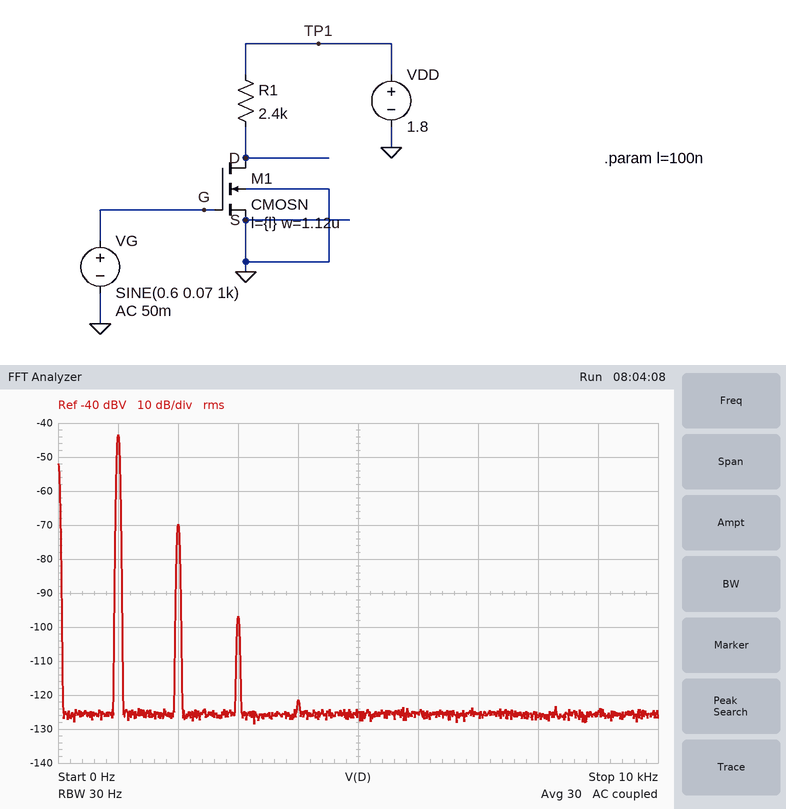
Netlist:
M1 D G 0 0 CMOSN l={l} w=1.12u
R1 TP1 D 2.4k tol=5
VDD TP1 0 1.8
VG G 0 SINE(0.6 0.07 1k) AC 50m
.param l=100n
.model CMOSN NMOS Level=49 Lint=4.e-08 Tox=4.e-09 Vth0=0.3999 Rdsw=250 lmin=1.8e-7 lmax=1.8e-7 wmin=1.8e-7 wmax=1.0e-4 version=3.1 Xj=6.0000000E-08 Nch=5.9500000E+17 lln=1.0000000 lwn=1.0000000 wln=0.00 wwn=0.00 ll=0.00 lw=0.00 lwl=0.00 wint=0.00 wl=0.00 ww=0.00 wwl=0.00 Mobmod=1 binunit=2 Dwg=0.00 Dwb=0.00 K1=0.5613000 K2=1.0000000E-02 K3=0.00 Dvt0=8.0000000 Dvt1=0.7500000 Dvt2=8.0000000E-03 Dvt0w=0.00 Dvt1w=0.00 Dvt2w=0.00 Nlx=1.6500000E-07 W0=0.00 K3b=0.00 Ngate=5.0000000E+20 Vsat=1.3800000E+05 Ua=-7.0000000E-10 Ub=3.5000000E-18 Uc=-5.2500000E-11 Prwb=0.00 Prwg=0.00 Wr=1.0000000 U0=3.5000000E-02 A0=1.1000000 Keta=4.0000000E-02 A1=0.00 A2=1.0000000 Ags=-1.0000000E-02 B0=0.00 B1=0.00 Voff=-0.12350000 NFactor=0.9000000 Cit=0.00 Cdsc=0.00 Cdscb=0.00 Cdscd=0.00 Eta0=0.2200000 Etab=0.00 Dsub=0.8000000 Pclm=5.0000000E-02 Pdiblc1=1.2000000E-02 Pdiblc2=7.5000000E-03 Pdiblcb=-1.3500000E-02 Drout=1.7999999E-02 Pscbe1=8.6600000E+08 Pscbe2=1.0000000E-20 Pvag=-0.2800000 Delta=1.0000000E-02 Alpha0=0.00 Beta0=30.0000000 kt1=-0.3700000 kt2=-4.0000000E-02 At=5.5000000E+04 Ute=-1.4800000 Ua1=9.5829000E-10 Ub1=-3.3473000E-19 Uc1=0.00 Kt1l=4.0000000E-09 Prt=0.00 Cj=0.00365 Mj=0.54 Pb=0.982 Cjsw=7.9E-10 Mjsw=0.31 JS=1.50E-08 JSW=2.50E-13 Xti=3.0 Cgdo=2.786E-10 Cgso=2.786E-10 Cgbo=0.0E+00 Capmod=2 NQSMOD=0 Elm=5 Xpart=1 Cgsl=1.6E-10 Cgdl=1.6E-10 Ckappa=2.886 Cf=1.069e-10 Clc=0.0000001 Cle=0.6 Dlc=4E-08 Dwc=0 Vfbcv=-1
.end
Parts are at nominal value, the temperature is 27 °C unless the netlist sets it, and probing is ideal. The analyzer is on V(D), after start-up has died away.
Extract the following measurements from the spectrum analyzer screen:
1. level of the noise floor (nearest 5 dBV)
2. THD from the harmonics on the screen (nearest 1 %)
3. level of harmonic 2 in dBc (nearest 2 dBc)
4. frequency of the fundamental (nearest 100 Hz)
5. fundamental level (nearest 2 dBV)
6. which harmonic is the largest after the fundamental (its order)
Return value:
-125 dBV
5 %
-26 dBc
1.0 kHz
-44 dBV
2
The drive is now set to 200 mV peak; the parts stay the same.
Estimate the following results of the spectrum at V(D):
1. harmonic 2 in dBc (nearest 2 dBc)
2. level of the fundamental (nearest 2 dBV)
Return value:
-18 dBc
-34 dBV
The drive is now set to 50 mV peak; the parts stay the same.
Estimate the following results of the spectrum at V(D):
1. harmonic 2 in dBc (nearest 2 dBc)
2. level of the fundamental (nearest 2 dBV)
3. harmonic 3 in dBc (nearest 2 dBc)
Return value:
-30 dBc
-46 dBV
-60 dBc
